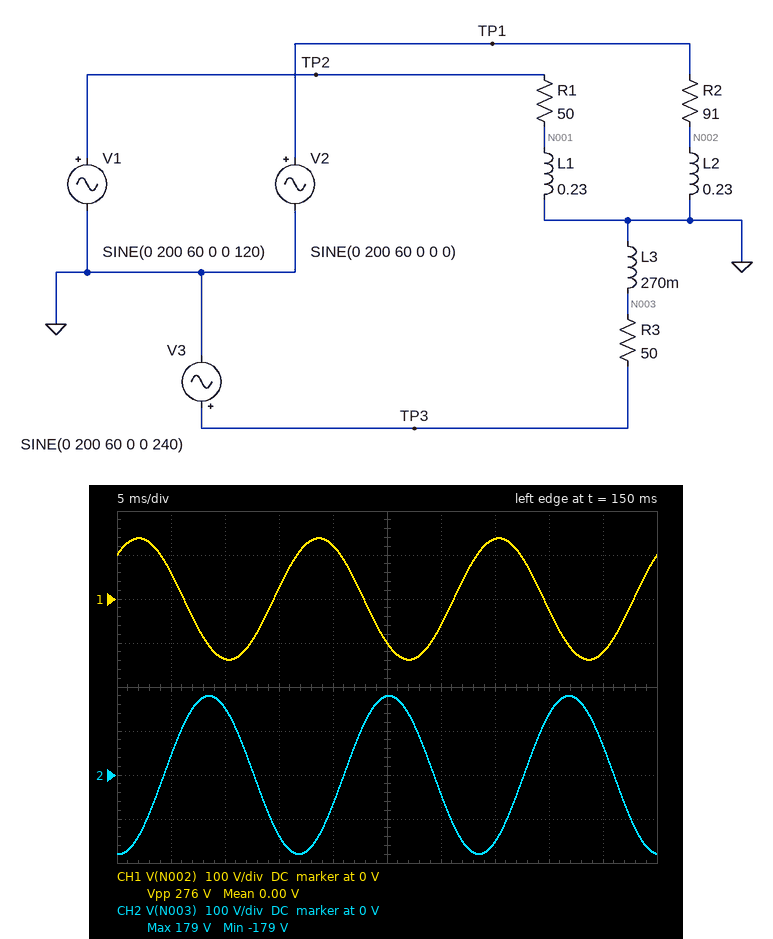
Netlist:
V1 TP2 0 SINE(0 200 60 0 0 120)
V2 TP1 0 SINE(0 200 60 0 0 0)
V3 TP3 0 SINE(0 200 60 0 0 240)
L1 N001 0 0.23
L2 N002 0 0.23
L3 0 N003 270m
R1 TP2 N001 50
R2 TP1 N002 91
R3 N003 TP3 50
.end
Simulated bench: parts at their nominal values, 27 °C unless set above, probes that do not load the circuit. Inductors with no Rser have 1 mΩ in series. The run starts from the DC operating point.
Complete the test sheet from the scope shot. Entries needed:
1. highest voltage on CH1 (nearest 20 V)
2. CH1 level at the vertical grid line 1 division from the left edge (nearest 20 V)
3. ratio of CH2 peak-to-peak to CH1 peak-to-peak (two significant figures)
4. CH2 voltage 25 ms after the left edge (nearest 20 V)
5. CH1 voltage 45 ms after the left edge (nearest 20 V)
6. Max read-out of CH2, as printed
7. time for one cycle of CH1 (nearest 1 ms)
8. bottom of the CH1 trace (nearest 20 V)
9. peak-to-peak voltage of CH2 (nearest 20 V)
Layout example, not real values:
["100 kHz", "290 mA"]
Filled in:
["140 V", "60 V", "1.3", "180 V", "-120 V", "179 V", "17 ms", "-140 V", "360 V"]
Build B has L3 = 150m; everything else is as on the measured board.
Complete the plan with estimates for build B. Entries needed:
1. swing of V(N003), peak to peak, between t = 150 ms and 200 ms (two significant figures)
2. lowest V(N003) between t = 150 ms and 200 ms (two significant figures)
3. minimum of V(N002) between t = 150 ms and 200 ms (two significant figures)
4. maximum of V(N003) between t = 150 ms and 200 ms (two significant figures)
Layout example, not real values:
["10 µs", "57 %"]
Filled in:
["300 V", "-150 V", "-140 V", "150 V"]
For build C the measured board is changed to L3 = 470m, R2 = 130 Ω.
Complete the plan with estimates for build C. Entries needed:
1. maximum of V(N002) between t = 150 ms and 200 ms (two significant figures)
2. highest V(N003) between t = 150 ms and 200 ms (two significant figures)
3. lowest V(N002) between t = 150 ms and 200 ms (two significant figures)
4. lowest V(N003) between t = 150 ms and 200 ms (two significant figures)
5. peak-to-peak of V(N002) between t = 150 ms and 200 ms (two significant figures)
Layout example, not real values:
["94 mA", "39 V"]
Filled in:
["110 V", "190 V", "-110 V", "-190 V", "220 V"]
